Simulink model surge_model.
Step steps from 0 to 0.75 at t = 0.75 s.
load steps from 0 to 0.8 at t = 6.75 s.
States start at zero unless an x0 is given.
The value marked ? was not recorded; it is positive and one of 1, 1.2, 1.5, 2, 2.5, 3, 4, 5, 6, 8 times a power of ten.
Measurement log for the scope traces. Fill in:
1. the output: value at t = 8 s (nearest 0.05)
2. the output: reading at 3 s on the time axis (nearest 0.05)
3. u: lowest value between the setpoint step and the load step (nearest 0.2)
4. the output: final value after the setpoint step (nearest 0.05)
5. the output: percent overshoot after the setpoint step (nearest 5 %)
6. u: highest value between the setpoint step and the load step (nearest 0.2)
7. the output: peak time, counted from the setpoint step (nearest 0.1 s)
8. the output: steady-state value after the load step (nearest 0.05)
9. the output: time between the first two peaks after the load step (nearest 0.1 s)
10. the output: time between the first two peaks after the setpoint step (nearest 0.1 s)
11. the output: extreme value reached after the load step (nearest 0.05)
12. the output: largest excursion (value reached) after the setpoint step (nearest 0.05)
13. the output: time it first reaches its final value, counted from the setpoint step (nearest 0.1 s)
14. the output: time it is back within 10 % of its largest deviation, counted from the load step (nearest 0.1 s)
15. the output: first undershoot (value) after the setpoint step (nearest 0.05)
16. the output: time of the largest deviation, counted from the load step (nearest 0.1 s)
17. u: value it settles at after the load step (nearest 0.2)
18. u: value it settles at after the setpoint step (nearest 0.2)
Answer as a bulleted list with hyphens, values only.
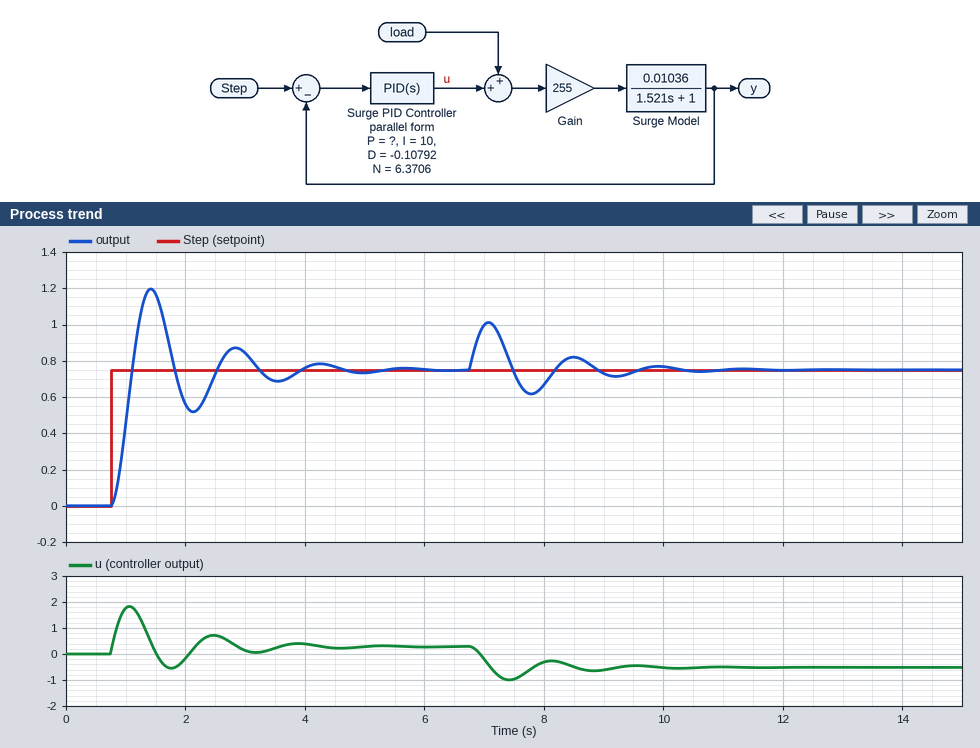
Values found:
- 0.65
- 0.85
- -0.6
- 0.75
- 60 %
- 1.8
- 0.7 s
- 0.75
- 1.4 s
- 1.4 s
- 1.00
- 1.20
- 0.4 s
- 2.6 s
- 0.50
- 0.3 s
- -0.6
- 0.2
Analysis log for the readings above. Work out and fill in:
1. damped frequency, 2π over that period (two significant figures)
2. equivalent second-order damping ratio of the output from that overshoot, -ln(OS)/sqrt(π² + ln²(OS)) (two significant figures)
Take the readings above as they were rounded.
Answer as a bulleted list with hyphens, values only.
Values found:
- 4.5 rad/s
- 0.16
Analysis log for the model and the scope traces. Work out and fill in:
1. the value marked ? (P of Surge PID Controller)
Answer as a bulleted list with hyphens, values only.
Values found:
- 0.8
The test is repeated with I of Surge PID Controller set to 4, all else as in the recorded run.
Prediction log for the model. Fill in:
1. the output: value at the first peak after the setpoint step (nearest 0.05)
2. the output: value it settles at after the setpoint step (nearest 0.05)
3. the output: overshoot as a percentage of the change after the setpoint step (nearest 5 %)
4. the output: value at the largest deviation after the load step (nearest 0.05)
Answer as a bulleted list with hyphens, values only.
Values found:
- 1.05
- 0.75
- 40 %
- 1.10
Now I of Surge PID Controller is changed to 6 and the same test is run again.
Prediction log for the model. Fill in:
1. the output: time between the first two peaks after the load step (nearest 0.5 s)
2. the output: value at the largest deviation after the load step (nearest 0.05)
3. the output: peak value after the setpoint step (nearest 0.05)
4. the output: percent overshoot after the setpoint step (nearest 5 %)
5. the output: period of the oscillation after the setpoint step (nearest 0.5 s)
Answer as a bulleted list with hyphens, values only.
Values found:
- 2.0 s
- 1.05
- 1.10
- 50 %
- 2.0 s
